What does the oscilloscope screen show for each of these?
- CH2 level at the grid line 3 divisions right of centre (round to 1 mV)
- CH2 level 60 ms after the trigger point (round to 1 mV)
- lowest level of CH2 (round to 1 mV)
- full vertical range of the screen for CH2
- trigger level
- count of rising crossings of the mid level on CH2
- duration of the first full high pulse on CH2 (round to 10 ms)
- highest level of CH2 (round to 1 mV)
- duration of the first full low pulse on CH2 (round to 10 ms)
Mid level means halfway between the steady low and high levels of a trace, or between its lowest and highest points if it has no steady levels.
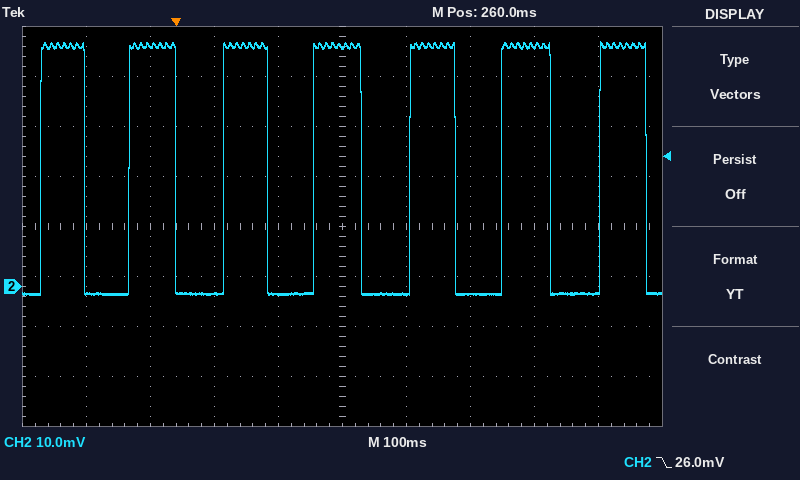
48 mV
-1 mV
-2 mV
80 mV
26.0 mV
7
70 ms
49 mV
70 ms
